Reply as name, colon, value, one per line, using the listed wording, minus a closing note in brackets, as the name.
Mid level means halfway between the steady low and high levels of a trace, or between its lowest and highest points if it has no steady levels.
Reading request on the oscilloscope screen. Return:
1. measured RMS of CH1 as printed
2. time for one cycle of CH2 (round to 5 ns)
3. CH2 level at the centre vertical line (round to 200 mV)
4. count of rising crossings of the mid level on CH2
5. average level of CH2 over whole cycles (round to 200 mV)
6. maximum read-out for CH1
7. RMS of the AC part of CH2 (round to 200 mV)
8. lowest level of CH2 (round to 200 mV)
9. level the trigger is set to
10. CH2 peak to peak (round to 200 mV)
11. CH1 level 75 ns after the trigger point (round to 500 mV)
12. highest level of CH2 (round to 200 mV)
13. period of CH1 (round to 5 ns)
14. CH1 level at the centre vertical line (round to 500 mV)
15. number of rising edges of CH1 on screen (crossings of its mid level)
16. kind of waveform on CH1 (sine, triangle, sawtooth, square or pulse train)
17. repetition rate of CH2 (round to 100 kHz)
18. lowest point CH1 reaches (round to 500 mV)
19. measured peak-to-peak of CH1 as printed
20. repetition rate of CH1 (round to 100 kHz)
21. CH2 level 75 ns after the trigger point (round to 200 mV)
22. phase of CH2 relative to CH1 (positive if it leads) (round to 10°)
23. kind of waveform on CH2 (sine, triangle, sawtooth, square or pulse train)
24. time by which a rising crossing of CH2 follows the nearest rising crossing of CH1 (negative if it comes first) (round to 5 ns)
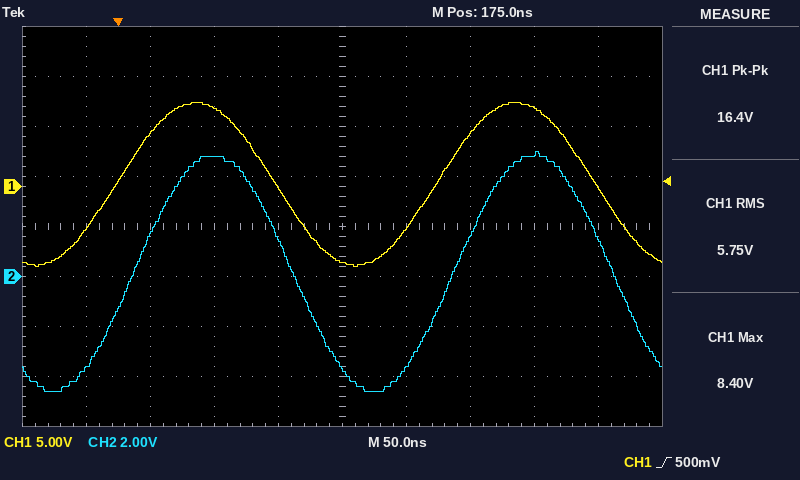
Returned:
measured RMS of CH1 as printed: 5.75 V
time for one cycle of CH2: 250 ns
CH2 level at the centre vertical line: -3.6 V
count of rising crossings of the mid level on CH2: 2
average level of CH2 over whole cycles: 200 mV
maximum read-out for CH1: 8.40 V
RMS of the AC part of CH2: 3.4 V
lowest level of CH2: -4.6 V
level the trigger is set to: 500 mV
CH2 peak to peak: 9.6 V
CH1 level 75 ns after the trigger point: 8.0 V
highest level of CH2: 5.0 V
period of CH1: 250 ns
CH1 level at the centre vertical line: -7.5 V
number of rising edges of CH1 on screen: 2
kind of waveform on CH1: sine
repetition rate of CH2: 4.0 MHz
lowest point CH1 reaches: -8.0 V
measured peak-to-peak of CH1 as printed: 16.4 V
repetition rate of CH1: 4.0 MHz
CH2 level 75 ns after the trigger point: 4.8 V
phase of CH2 relative to CH1 (positive if it leads): -20°
kind of waveform on CH2: sine
time by which a rising crossing of CH2 follows the nearest rising crossing of CH1 (negative if it comes first): +15 ns
